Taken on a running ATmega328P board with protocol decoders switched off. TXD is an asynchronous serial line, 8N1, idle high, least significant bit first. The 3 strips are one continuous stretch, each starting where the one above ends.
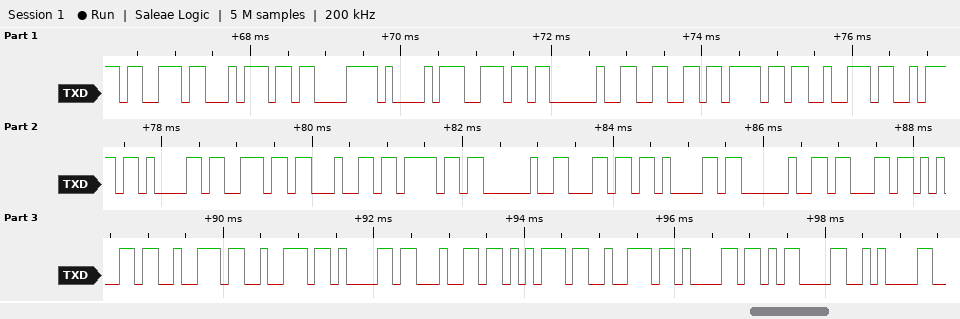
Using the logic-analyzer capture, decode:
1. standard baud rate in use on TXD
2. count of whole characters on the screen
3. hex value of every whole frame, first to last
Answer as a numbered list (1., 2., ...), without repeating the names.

1. 9600 baud
2. 29
3. 73 74 C3 A1 6E 20 66 6F 72 7A 61 6E 64 6F 20 6C 61 20 63 65 72 72 61 64 75 72 61 0D 0A
